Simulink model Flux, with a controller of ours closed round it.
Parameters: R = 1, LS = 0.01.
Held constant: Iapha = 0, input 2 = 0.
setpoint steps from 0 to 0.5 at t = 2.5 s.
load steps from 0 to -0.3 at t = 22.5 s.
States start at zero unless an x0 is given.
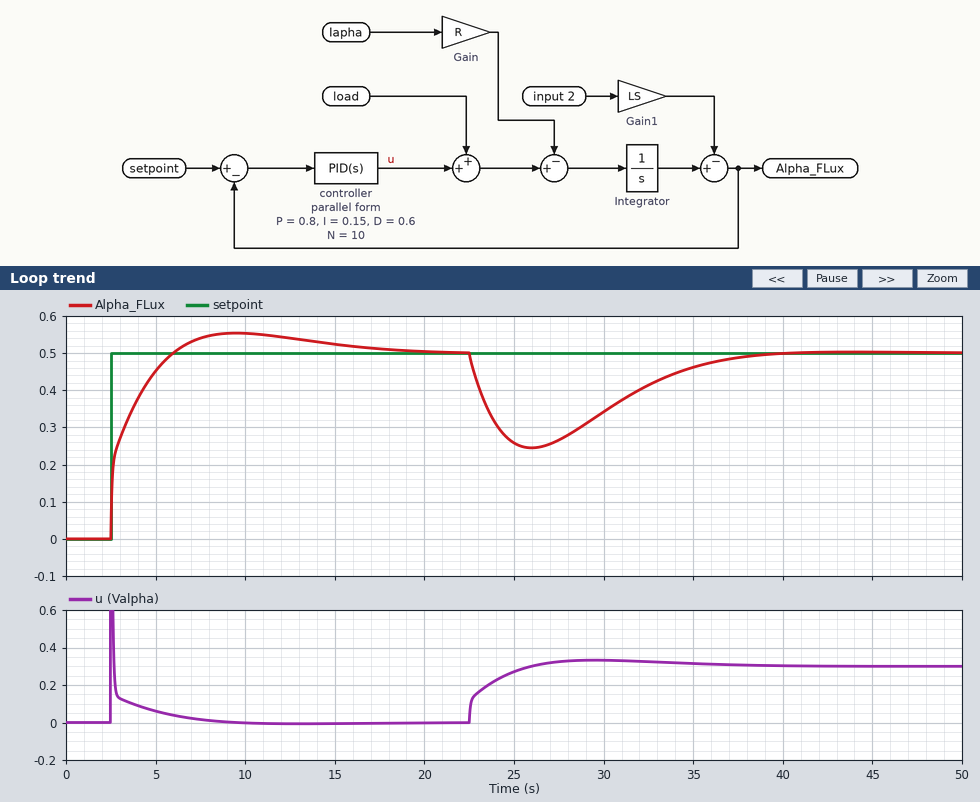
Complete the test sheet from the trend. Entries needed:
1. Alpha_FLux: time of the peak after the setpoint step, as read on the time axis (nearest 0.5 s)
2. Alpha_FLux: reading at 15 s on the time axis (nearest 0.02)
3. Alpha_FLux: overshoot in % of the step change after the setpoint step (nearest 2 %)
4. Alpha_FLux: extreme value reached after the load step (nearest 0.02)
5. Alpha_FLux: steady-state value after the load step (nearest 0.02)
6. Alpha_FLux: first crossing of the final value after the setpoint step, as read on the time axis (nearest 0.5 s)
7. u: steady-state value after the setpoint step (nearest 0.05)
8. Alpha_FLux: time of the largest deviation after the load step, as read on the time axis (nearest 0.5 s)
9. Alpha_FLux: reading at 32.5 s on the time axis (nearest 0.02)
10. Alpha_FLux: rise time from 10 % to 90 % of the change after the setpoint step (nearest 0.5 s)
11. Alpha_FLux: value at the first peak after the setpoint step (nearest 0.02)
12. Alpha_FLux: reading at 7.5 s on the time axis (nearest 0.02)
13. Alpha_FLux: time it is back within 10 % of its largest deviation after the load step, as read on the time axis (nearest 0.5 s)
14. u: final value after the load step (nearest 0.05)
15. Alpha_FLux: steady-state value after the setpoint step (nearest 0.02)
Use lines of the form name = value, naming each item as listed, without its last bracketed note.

Alpha_FLux: time of the peak after the setpoint step, as read on the time axis = 9.5 s
Alpha_FLux: reading at 15 s on the time axis = 0.52
Alpha_FLux: overshoot in % of the step change after the setpoint step = 10 %
Alpha_FLux: extreme value reached after the load step = 0.24
Alpha_FLux: steady-state value after the load step = 0.50
Alpha_FLux: first crossing of the final value after the setpoint step, as read on the time axis = 6.0 s
u: steady-state value after the setpoint step = 0.00
Alpha_FLux: time of the largest deviation after the load step, as read on the time axis = 26.0 s
Alpha_FLux: reading at 32.5 s on the time axis = 0.42
Alpha_FLux: rise time from 10 % to 90 % of the change after the setpoint step = 2.5 s
Alpha_FLux: value at the first peak after the setpoint step = 0.56
Alpha_FLux: reading at 7.5 s on the time axis = 0.54
Alpha_FLux: time it is back within 10 % of its largest deviation after the load step, as read on the time axis = 36.0 s
u: final value after the load step = 0.30
Alpha_FLux: steady-state value after the setpoint step = 0.50
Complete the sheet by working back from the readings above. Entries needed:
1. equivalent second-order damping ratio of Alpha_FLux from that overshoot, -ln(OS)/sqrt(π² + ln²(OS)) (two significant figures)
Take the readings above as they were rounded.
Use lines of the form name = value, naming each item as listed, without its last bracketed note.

equivalent second-order damping ratio of Alpha_FLux from that overshoot, -ln(OS)/sqrt(π² + ln²(OS)) = 0.59
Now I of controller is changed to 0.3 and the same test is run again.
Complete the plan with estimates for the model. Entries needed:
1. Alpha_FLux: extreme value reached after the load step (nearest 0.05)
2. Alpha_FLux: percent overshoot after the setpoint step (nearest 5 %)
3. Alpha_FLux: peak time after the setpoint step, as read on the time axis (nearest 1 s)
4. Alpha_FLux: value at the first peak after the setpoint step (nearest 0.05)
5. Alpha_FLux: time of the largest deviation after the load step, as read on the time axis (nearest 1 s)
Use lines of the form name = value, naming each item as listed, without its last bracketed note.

Alpha_FLux: extreme value reached after the load step = 0.30
Alpha_FLux: percent overshoot after the setpoint step = 15 %
Alpha_FLux: peak time after the setpoint step, as read on the time axis = 8 s
Alpha_FLux: value at the first peak after the setpoint step = 0.60
Alpha_FLux: time of the largest deviation after the load step, as read on the time axis = 25 s
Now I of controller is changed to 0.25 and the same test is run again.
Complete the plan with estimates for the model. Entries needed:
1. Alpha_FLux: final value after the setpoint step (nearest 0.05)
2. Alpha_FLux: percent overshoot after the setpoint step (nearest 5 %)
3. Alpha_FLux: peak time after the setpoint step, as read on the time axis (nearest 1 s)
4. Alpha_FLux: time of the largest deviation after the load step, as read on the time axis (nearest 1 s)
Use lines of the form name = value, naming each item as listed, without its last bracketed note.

Alpha_FLux: final value after the setpoint step = 0.50
Alpha_FLux: percent overshoot after the setpoint step = 15 %
Alpha_FLux: peak time after the setpoint step, as read on the time axis = 8 s
Alpha_FLux: time of the largest deviation after the load step, as read on the time axis = 25 s
